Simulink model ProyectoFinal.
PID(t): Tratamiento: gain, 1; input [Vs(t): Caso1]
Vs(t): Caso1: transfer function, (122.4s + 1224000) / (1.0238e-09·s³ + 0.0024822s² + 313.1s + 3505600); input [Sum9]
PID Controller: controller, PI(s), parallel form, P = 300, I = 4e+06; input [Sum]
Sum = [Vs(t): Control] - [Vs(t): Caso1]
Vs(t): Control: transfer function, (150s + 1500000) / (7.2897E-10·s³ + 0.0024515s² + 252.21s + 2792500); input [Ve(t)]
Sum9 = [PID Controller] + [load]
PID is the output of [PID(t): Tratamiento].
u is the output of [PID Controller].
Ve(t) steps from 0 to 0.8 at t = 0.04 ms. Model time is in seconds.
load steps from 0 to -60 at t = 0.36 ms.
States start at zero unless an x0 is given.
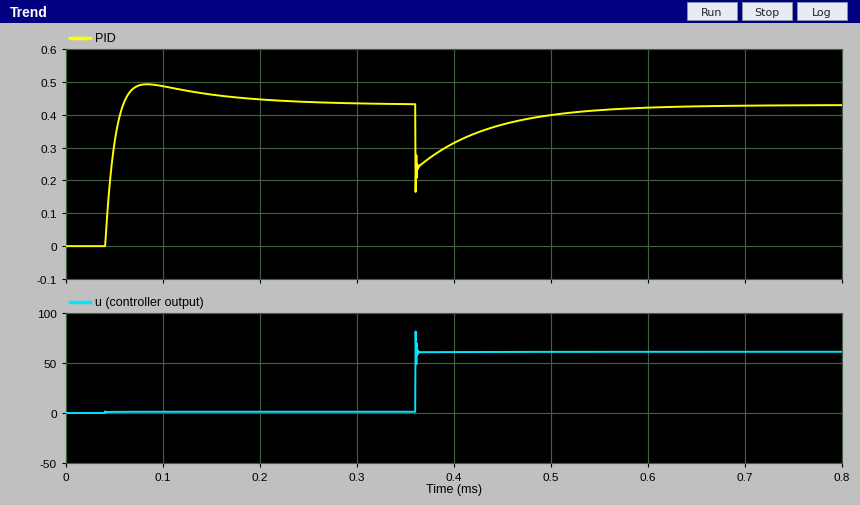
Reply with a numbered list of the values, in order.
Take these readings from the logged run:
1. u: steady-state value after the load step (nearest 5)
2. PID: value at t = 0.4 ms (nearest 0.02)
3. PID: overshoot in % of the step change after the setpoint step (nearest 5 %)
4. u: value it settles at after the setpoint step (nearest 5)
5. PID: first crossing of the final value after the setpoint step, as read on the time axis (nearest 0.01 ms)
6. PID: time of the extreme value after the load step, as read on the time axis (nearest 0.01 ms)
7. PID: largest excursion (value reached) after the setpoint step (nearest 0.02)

1. 60
2. 0.32
3. 15 %
4. 0
5. 0.06 ms
6. 0.36 ms
7. 0.50
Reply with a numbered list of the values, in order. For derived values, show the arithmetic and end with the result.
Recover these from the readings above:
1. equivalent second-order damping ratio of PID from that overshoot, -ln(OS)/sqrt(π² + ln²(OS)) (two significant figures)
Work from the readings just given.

1. ln(0.15) = -1.897; 1.897 / sqrt(9.870 + 3.599) = 0.52
